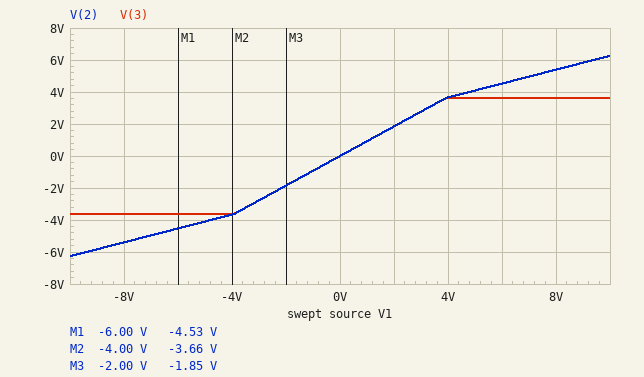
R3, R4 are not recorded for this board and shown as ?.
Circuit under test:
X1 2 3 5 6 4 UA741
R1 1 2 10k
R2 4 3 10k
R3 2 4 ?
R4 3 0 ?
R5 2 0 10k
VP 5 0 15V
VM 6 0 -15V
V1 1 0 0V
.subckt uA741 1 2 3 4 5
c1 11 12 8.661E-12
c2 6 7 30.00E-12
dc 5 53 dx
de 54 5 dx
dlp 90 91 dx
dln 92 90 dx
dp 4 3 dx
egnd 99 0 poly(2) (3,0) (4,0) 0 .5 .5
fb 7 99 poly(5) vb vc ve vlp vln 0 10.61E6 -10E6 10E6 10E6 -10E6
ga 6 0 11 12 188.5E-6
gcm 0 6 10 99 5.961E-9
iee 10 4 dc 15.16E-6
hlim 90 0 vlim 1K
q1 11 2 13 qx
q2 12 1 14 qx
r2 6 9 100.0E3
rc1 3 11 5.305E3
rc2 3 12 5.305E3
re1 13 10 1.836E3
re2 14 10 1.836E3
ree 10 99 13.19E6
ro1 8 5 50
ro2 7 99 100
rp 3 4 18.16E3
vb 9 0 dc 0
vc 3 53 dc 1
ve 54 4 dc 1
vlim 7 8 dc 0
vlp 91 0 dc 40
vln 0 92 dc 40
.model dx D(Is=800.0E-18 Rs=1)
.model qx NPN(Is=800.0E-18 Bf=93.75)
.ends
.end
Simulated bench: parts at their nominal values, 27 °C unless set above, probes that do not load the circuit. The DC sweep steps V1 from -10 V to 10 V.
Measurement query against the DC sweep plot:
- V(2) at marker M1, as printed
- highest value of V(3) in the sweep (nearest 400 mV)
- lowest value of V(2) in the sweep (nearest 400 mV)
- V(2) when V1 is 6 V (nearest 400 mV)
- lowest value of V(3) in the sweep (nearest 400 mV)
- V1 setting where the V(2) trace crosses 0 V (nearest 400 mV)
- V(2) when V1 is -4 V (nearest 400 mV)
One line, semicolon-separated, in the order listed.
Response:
-4.53 V; 3.6 V; -6.4 V; 4.4 V; -3.6 V; 0 V; -3.6 V
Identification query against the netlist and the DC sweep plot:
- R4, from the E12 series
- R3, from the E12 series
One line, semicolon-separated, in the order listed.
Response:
3.3 kΩ; 33 kΩ
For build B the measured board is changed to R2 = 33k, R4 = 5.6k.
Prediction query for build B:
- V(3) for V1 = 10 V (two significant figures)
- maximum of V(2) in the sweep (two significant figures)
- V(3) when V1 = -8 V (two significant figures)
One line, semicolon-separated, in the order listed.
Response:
2.1 V; 6.3 V; -2.1 V
